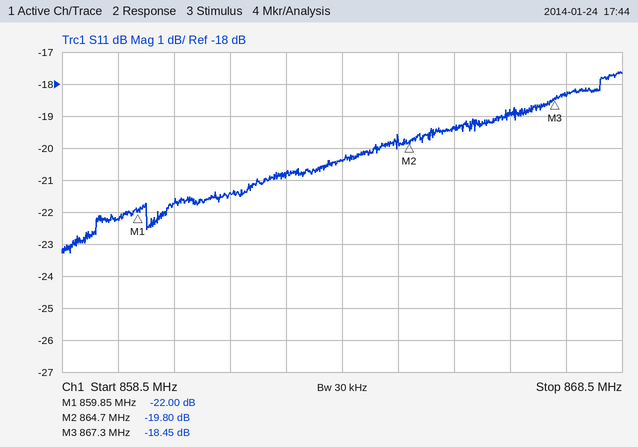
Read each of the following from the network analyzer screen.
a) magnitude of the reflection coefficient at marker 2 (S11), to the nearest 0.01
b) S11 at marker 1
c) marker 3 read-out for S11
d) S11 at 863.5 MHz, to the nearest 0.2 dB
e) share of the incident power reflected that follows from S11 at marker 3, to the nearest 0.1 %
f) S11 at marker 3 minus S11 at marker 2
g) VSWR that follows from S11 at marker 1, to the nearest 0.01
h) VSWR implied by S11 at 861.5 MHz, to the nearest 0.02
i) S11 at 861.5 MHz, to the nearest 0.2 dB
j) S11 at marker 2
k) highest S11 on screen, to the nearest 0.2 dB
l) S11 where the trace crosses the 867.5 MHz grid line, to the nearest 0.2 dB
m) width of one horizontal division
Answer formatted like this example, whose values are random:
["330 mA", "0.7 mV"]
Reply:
["0.10", "-22.00 dB", "-18.45 dB", "-20.4 dB", "1.4 %", "1.35 dB", "1.17", "1.18", "-21.4 dB", "-19.80 dB", "-17.6 dB", "-18.4 dB", "1 MHz"]
